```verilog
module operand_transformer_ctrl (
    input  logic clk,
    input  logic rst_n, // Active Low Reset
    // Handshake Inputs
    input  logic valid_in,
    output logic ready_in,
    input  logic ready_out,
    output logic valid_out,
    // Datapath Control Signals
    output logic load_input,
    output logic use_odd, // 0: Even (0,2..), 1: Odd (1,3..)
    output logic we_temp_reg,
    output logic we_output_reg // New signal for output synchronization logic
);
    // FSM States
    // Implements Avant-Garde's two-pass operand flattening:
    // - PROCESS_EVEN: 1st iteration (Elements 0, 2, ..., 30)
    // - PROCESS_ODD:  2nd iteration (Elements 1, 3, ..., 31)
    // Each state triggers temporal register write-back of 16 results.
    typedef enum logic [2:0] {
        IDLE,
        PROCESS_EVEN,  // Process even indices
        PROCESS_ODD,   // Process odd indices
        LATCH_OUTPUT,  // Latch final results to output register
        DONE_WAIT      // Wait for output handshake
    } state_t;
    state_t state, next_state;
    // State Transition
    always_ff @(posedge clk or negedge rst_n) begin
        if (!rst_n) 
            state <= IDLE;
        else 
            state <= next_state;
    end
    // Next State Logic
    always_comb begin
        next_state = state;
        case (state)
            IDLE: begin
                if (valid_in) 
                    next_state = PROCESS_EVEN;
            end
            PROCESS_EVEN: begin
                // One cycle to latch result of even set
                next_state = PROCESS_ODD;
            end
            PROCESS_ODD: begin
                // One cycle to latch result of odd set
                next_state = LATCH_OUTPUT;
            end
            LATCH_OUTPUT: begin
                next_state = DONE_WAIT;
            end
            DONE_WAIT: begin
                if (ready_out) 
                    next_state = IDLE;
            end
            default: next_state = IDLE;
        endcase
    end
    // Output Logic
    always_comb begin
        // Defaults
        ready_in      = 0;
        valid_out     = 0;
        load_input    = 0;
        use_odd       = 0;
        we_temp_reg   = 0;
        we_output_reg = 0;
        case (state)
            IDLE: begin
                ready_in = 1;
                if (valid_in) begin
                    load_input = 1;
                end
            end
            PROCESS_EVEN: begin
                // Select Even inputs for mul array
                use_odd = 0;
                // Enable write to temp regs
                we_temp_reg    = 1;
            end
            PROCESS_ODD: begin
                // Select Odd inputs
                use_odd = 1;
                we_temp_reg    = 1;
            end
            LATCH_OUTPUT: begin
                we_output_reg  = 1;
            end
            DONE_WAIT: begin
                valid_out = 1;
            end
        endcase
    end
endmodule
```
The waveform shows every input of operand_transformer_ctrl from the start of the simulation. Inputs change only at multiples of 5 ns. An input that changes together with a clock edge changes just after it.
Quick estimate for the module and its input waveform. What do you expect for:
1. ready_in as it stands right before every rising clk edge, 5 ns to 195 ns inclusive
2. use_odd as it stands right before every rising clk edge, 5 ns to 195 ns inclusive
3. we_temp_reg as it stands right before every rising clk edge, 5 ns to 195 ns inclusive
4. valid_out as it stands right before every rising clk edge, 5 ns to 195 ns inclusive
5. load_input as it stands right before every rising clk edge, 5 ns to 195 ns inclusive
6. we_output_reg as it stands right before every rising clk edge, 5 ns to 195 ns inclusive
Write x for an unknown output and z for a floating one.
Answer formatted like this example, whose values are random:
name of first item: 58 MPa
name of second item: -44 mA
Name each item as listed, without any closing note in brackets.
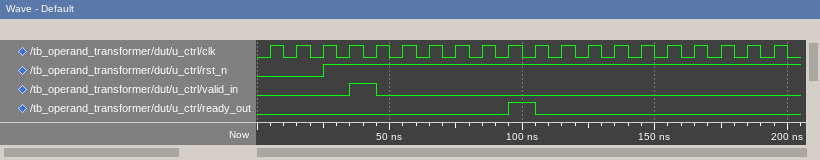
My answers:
ready_in as it stands right before every rising clk edge, 5 ns to 195 ns inclusive: 1 1 1 1 1 0 0 0 0 0 0 1 1 1 1 1 1 1 1 1
use_odd as it stands right before every rising clk edge, 5 ns to 195 ns inclusive: 0 0 0 0 0 0 1 0 0 0 0 0 0 0 0 0 0 0 0 0
we_temp_reg as it stands right before every rising clk edge, 5 ns to 195 ns inclusive: 0 0 0 0 0 1 1 0 0 0 0 0 0 0 0 0 0 0 0 0
valid_out as it stands right before every rising clk edge, 5 ns to 195 ns inclusive: 0 0 0 0 0 0 0 0 1 1 1 0 0 0 0 0 0 0 0 0
load_input as it stands right before every rising clk edge, 5 ns to 195 ns inclusive: 0 0 0 0 1 0 0 0 0 0 0 0 0 0 0 0 0 0 0 0
we_output_reg as it stands right before every rising clk edge, 5 ns to 195 ns inclusive: 0 0 0 0 0 0 0 1 0 0 0 0 0 0 0 0 0 0 0 0
